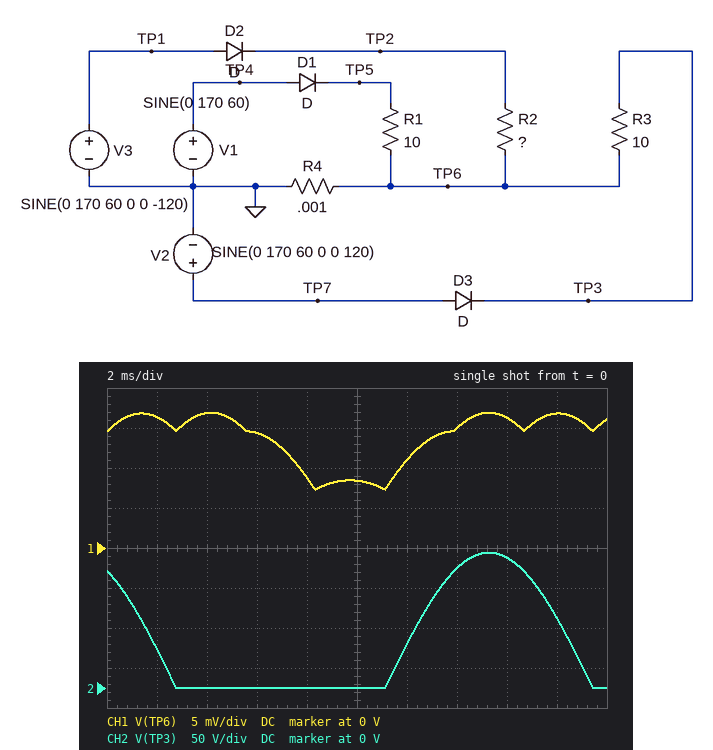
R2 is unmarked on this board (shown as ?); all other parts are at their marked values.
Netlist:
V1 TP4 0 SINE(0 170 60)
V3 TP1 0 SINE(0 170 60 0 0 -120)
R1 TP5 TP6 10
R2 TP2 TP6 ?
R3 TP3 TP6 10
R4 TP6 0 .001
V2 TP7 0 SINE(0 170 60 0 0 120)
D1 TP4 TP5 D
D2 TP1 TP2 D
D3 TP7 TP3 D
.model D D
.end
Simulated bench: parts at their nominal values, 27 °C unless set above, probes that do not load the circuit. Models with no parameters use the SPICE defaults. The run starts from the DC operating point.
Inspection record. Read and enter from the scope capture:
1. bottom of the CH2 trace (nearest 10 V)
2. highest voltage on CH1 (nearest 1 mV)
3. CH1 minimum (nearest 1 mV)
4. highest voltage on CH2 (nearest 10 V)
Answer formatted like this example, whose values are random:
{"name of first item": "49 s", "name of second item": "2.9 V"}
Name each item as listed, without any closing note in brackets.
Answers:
{"bottom of the CH2 trace": "0 V", "highest voltage on CH1": "17 mV", "CH1 minimum": "7 mV", "highest voltage on CH2": "170 V"}
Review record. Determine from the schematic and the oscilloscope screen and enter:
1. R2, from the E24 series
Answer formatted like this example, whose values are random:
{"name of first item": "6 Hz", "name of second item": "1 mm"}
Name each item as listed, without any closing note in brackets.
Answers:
{"R2, from the E24 series": "20 Ω"}
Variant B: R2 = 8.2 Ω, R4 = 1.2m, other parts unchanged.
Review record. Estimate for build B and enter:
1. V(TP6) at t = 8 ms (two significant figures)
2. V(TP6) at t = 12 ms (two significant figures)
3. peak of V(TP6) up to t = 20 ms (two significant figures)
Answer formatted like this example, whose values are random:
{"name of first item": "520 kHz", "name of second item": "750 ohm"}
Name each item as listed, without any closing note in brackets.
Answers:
{"V(TP6) at t = 8 ms": "22 mV", "V(TP6) at t = 12 ms": "23 mV", "peak of V(TP6) up to t = 20 ms": "25 mV"}
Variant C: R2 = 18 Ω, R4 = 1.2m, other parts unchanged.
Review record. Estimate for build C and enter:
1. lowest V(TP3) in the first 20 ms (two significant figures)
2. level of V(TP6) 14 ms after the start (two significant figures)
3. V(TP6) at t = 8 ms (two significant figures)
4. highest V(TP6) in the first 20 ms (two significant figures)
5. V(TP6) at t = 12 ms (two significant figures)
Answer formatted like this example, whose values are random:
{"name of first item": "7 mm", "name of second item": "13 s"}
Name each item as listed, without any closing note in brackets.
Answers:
{"lowest V(TP3) in the first 20 ms": "9.7 mV", "level of V(TP6) 14 ms after the start": "18 mV", "V(TP6) at t = 8 ms": "11 mV", "highest V(TP6) in the first 20 ms": "20 mV", "V(TP6) at t = 12 ms": "14 mV"}
